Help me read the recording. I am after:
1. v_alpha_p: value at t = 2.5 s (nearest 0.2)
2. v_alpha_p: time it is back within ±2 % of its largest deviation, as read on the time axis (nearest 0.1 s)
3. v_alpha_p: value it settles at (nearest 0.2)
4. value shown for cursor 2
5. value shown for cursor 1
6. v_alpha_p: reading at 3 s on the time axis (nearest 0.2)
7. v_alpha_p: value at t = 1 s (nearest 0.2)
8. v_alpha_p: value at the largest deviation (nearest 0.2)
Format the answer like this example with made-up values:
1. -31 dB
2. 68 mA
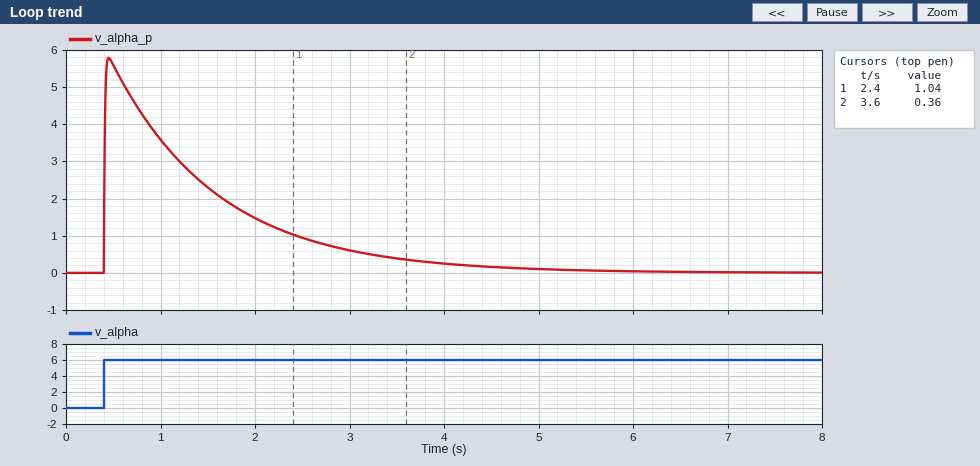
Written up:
1. 1.0
2. 4.9 s
3. 0.0
4. 0.36
5. 1.04
6. 0.6
7. 3.6
8. 5.8
